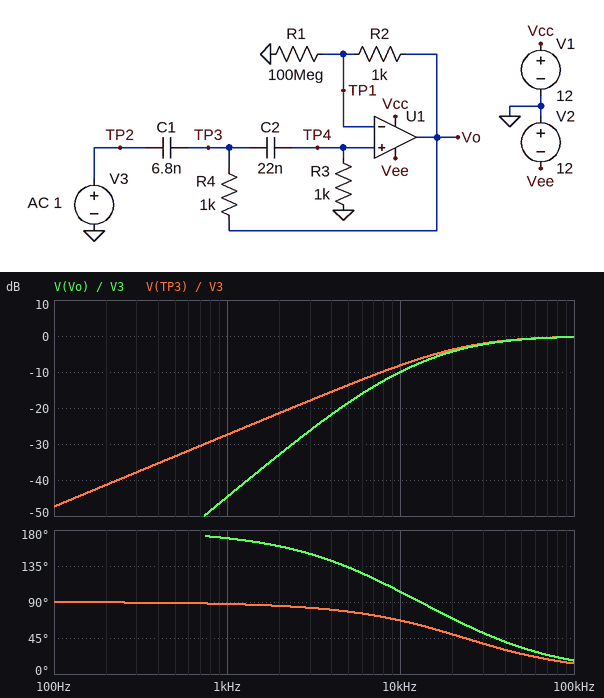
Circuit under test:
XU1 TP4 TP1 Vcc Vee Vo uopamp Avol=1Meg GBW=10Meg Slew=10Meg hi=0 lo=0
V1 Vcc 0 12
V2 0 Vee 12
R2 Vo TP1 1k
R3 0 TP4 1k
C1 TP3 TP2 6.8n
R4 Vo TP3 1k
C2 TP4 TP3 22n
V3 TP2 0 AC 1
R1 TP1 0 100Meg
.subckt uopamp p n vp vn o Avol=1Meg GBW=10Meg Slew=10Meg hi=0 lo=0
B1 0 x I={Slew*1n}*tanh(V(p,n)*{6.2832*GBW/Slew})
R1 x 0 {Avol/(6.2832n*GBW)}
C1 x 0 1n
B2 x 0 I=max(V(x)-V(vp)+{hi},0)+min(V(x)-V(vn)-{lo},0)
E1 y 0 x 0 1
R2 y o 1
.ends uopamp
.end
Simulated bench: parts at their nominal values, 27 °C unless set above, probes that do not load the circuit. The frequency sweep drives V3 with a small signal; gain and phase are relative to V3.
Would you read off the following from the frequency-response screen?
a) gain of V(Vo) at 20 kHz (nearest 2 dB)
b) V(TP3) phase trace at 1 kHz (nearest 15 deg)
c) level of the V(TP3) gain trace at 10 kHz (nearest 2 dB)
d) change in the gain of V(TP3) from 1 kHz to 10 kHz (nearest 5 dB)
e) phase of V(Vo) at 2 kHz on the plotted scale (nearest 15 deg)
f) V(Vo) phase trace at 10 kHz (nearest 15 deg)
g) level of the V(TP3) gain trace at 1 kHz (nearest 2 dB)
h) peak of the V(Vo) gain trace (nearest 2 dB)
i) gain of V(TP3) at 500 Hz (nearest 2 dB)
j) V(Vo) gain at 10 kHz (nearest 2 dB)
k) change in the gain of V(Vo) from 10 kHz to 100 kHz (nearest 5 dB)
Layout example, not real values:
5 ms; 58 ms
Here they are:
-4 dB; 90 deg; -8 dB; 20 dB; 165 deg; 105 deg; -28 dB; 0 dB; -34 dB; -10 dB; 10 dB
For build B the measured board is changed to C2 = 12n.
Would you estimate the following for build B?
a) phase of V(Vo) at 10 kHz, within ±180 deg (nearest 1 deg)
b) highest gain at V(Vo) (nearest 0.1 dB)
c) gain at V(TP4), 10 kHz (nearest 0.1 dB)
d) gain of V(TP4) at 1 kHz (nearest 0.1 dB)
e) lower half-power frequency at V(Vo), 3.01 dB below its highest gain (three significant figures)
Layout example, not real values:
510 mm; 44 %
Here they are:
120 deg; 0 dB; -12.5 dB; -49.9 dB; 28.7 kHz
